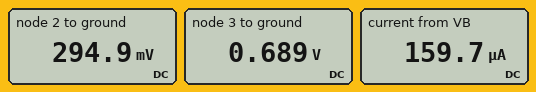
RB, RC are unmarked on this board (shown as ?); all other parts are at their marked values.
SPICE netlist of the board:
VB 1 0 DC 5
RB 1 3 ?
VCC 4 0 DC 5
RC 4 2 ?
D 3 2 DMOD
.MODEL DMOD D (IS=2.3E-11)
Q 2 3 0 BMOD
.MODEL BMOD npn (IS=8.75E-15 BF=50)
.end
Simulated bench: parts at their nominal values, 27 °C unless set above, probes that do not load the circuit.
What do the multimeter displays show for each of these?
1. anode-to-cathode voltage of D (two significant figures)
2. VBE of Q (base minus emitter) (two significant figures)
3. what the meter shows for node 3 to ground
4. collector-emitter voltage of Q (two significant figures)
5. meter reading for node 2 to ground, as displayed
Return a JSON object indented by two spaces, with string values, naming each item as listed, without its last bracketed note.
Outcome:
{
  "anode-to-cathode voltage of D": "390 mV",
  "VBE of Q (base minus emitter)": "690 mV",
  "what the meter shows for node 3 to ground": "0.689 V",
  "collector-emitter voltage of Q": "290 mV",
  "meter reading for node 2 to ground, as displayed": "294.9 mV"
}
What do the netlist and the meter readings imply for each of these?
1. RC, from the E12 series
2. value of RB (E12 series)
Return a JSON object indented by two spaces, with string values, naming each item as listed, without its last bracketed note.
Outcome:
{
  "RC, from the E12 series": "1.5 kΩ",
  "value of RB": "27 kΩ"
}
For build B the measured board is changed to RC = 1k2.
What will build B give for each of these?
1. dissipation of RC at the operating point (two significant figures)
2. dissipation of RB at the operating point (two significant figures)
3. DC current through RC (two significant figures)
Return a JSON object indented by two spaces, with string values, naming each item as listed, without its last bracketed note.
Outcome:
{
  "dissipation of RC at the operating point": "18 mW",
  "dissipation of RB at the operating point": "690 µW",
  "DC current through RC": "3.9 mA"
}
